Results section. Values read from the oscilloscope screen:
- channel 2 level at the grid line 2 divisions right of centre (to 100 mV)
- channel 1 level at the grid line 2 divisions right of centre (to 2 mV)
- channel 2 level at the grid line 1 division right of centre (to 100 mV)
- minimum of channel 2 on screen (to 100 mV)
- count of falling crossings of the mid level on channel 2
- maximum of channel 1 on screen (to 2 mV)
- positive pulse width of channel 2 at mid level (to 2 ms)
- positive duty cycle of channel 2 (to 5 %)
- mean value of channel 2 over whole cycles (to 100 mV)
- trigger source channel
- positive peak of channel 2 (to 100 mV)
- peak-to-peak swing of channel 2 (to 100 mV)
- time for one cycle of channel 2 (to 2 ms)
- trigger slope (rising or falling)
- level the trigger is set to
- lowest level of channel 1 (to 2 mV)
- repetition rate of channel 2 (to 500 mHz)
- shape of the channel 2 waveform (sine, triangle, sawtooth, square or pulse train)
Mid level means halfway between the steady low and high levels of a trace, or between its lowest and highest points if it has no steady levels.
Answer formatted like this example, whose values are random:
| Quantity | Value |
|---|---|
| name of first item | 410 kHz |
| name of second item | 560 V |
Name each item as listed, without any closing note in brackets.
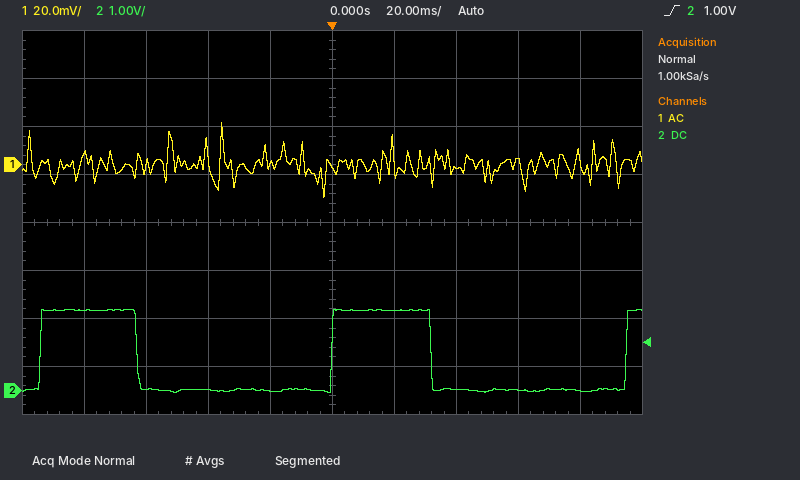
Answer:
| Quantity | Value |
|---|---|
| channel 2 level at the grid line 2 divisions right of centre | 0.0 V |
| channel 1 level at the grid line 2 divisions right of centre | -2 mV |
| channel 2 level at the grid line 1 division right of centre | 1.7 V |
| minimum of channel 2 on screen | 0.0 V |
| count of falling crossings of the mid level on channel 2 | 2 |
| maximum of channel 1 on screen | 18 mV |
| positive pulse width of channel 2 at mid level | 32 ms |
| positive duty cycle of channel 2 | 35 % |
| mean value of channel 2 over whole cycles | 600 mV |
| trigger source channel | channel 2 |
| positive peak of channel 2 | 1.7 V |
| peak-to-peak swing of channel 2 | 1.7 V |
| time for one cycle of channel 2 | 94 ms |
| trigger slope | rising |
| level the trigger is set to | 1.00 V |
| lowest level of channel 1 | -14 mV |
| repetition rate of channel 2 | 10.5 Hz |
| shape of the channel 2 waveform | pulse train |
